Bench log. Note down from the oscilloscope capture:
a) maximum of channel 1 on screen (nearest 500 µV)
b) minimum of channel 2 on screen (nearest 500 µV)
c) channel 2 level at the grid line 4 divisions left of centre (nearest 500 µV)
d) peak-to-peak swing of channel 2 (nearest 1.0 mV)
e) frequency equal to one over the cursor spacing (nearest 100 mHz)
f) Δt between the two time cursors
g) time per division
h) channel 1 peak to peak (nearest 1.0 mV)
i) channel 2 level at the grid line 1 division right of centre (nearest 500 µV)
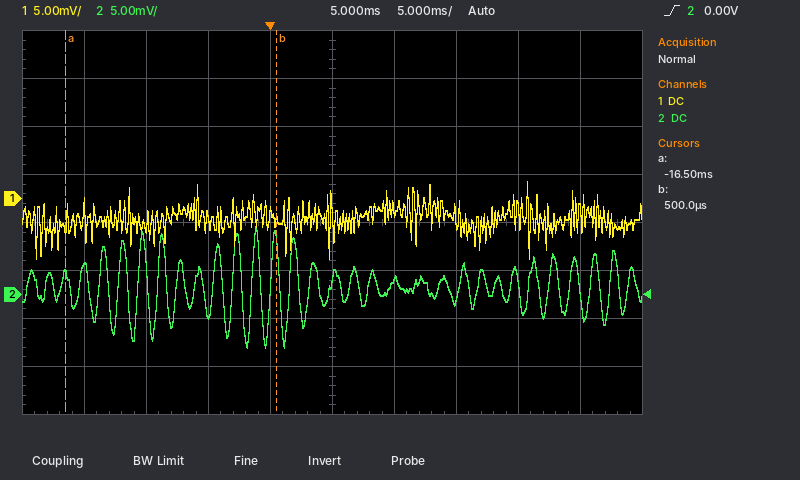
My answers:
2.0 mV
-5.5 mV
3.0 mV
13.0 mV
58.8 Hz
17.0 ms
5 ms
8.0 mV
1.5 mV
